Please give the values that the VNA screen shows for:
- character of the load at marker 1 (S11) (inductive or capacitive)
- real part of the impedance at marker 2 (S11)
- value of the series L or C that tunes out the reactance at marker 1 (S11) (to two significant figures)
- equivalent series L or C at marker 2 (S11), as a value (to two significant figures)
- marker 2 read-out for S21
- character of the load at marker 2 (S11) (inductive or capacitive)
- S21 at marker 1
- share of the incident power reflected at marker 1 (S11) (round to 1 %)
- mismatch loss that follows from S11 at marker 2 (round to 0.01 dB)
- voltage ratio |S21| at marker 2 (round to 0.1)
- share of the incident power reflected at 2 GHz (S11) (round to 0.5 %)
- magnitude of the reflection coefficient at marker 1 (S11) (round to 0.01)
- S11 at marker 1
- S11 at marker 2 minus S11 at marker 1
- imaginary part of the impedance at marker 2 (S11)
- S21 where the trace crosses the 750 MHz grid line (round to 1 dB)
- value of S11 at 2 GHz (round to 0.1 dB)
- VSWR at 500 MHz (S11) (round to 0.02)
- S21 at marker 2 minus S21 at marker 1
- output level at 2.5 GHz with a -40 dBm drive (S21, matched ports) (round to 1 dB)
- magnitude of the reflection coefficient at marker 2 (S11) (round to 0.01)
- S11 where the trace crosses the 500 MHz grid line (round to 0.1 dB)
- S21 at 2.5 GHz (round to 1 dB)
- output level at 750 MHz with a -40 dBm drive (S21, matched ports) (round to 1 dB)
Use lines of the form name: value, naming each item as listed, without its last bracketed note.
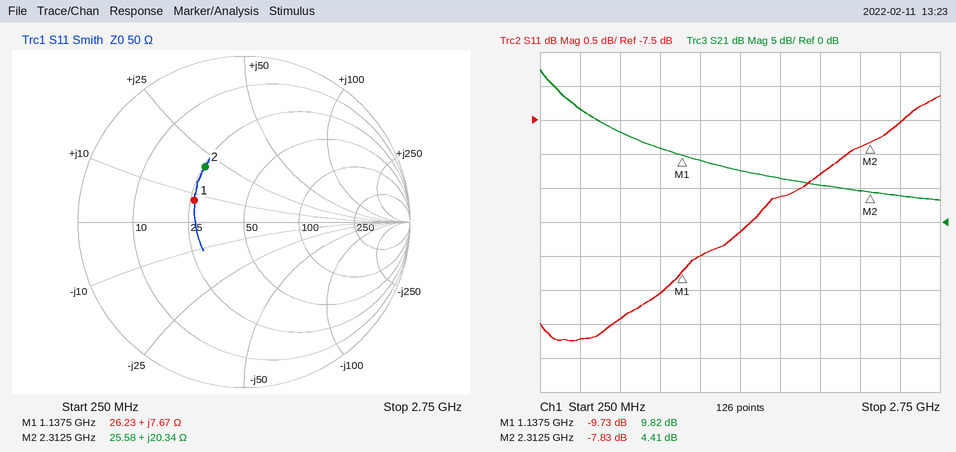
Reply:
character of the load at marker 1 (S11): inductive
real part of the impedance at marker 2: 25.58 Ω
value of the series L or C that tunes out the reactance at marker 1 (S11): 18 pF
equivalent series L or C at marker 2 (S11), as a value: 1.4 nH
marker 2 read-out for S21: 4.41 dB
character of the load at marker 2 (S11): inductive
S21 at marker 1: 9.82 dB
share of the incident power reflected at marker 1 (S11): 11 %
mismatch loss that follows from S11 at marker 2: 0.78 dB
voltage ratio |S21| at marker 2: 1.7
share of the incident power reflected at 2 GHz (S11): 15.0 %
magnitude of the reflection coefficient at marker 1 (S11): 0.33
S11 at marker 1: -9.73 dB
S11 at marker 2 minus S11 at marker 1: 1.90 dB
imaginary part of the impedance at marker 2: +20.34 Ω
S21 where the trace crosses the 750 MHz grid line: 13 dB
value of S11 at 2 GHz: -8.3 dB
VSWR at 500 MHz (S11): 1.82
S21 at marker 2 minus S21 at marker 1: -5.41 dB
output level at 2.5 GHz with a -40 dBm drive (S21, matched ports): -36 dBm
magnitude of the reflection coefficient at marker 2 (S11): 0.41
S11 where the trace crosses the 500 MHz grid line: -10.7 dB
S21 at 2.5 GHz: 4 dB
output level at 750 MHz with a -40 dBm drive (S21, matched ports): -27 dBm
